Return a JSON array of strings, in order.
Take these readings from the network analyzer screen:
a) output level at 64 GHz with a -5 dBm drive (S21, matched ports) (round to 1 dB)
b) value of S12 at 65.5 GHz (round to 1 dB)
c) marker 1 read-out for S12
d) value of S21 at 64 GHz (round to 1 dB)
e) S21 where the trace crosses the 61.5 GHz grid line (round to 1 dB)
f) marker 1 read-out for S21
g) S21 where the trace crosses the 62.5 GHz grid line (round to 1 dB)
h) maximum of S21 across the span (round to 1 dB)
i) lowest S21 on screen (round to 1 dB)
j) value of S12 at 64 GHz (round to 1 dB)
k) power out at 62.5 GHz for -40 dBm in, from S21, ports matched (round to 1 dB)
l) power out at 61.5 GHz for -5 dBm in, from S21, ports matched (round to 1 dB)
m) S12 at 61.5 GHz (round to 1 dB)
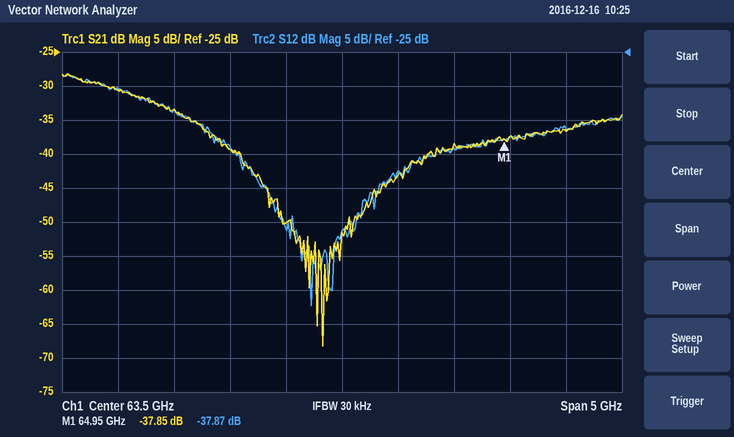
["-48 dBm", "-36 dB", "-37.87 dB", "-43 dB", "-31 dB", "-37.85 dB", "-39 dB", "-28 dB", "-68 dB", "-43 dB", "-79 dBm", "-36 dBm", "-30 dB"]
